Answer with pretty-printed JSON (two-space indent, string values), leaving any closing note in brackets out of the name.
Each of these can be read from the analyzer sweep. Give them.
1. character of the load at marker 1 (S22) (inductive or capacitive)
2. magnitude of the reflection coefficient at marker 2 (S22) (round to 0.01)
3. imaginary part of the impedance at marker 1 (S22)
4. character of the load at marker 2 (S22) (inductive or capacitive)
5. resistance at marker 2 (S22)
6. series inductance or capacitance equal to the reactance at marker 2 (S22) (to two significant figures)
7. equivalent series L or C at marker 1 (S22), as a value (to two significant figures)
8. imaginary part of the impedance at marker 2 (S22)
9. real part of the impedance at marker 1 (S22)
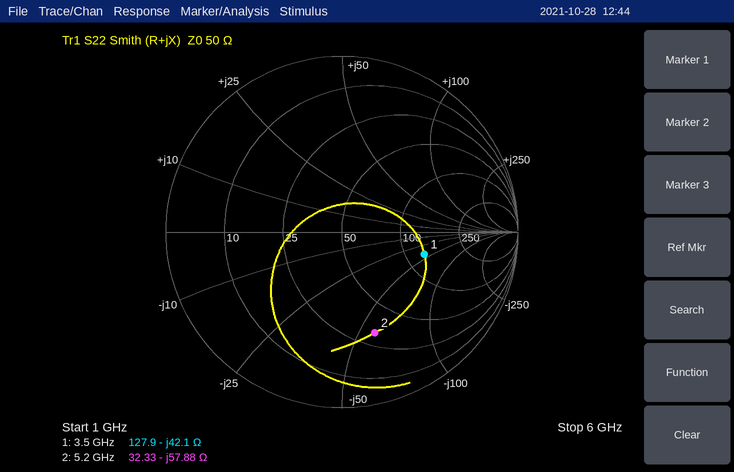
{
  "character of the load at marker 1 (S22)": "capacitive",
  "magnitude of the reflection coefficient at marker 2 (S22)": "0.60",
  "imaginary part of the impedance at marker 1": "-42.1 Ω",
  "character of the load at marker 2 (S22)": "capacitive",
  "resistance at marker 2": "32.33 Ω",
  "series inductance or capacitance equal to the reactance at marker 2 (S22)": "530 fF",
  "equivalent series L or C at marker 1 (S22), as a value": "1.1 pF",
  "imaginary part of the impedance at marker 2": "-57.88 Ω",
  "real part of the impedance at marker 1": "127.9 Ω"
}
